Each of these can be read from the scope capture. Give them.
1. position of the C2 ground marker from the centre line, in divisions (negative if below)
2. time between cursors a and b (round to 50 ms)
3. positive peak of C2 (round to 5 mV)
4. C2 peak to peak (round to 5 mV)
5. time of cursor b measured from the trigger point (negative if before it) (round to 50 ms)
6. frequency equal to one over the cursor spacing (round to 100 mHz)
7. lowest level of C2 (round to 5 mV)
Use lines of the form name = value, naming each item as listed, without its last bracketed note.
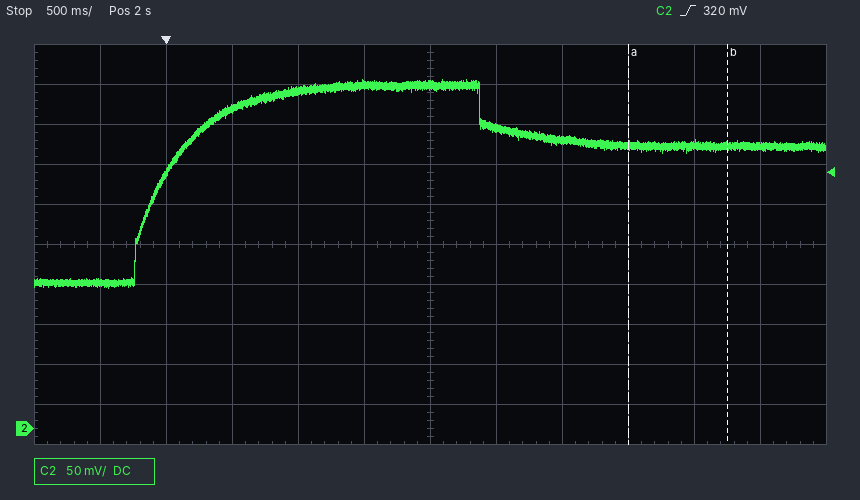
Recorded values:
position of the C2 ground marker from the centre line, in divisions = -4.6 div
time between cursors a and b = 750 ms
positive peak of C2 = 435 mV
C2 peak to peak = 260 mV
time of cursor b measured from the trigger point (negative if before it) = +4.25 s
frequency equal to one over the cursor spacing = 1.3 Hz
lowest level of C2 = 175 mV
